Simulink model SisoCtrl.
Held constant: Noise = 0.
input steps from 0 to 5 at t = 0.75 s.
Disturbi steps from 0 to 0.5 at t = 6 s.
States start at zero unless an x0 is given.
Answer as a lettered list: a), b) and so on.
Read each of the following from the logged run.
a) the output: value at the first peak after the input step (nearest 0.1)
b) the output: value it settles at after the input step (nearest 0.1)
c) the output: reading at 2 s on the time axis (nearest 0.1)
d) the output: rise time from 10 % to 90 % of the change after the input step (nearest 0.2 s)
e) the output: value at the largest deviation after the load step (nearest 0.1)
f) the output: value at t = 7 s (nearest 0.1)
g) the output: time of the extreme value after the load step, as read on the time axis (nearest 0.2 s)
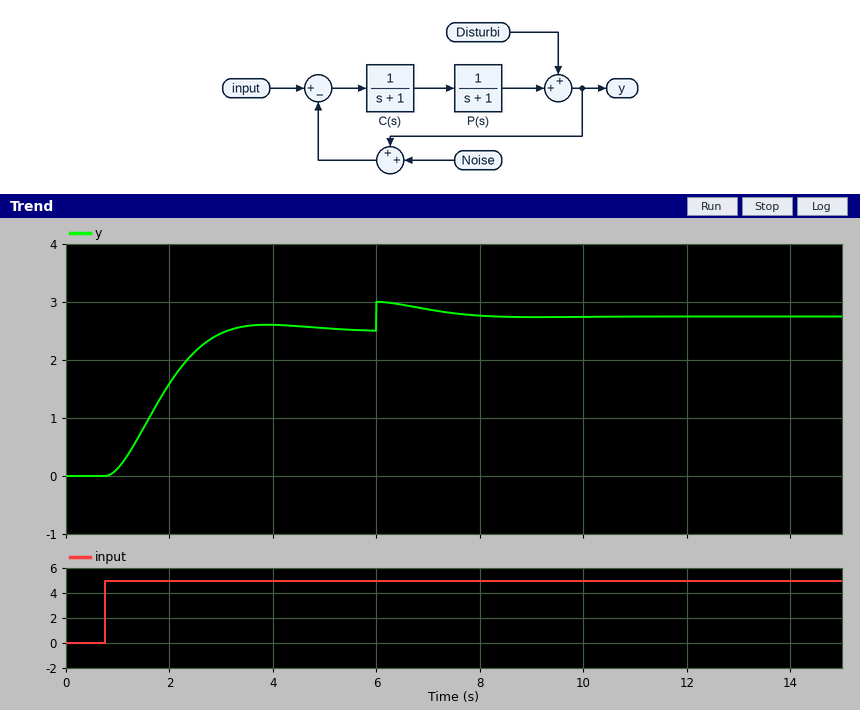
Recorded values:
a) 2.6
b) 2.5
c) 1.6
d) 1.6 s
e) 3.0
f) 2.9
g) 6.0 s
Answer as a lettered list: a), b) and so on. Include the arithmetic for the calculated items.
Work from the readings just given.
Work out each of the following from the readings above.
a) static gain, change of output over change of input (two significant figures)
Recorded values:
a) (2.5 - 0) / (5 - 0) = 0.50
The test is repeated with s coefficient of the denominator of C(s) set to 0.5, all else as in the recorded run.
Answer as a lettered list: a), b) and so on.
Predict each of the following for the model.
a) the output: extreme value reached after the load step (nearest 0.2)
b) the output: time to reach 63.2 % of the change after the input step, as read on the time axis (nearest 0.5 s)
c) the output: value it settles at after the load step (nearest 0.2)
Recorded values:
a) 3.0
b) 1.5 s
c) 2.8
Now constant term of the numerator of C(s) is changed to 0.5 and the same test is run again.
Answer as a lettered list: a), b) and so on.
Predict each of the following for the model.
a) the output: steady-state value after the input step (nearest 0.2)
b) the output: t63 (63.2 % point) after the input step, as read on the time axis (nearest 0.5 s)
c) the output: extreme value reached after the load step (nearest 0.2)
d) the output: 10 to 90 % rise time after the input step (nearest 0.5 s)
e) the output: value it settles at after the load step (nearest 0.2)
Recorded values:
a) 1.6
b) 2.5 s
c) 2.2
d) 2.0 s
e) 2.0
